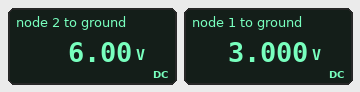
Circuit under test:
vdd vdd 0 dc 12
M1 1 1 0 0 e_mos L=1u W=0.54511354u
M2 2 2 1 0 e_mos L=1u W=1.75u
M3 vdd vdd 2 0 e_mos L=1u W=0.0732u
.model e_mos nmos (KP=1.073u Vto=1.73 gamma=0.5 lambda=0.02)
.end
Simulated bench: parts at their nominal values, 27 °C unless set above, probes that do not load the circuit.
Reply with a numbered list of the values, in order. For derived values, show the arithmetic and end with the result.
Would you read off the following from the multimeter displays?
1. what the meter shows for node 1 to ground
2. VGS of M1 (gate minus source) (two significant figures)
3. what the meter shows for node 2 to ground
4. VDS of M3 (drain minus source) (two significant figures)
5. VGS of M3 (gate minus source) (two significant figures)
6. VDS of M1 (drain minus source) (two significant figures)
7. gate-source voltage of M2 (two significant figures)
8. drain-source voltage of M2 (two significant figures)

1. 3.000 V
2. 3 V = 3.0 V
3. 6.00 V
4. 12 V - 6 V = 6.0 V
5. 12 V - 6 V = 6.0 V
6. 3 V = 3.0 V
7. 6 V - 3 V = 3.0 V
8. 6 V - 3 V = 3.0 V
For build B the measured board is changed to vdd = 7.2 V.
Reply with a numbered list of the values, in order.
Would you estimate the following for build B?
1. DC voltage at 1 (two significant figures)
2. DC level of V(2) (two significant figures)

1. 1.9 V
2. 4.2 V
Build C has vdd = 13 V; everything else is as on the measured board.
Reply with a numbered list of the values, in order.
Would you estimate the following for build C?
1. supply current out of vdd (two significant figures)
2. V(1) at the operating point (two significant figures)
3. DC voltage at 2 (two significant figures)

1. 700 nA
2. 3.2 V
3. 6.4 V
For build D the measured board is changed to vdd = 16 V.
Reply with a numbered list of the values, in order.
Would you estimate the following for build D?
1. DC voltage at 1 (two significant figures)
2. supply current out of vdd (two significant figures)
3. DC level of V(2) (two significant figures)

1. 3.9 V
2. 1.5 µA
3. 7.5 V
